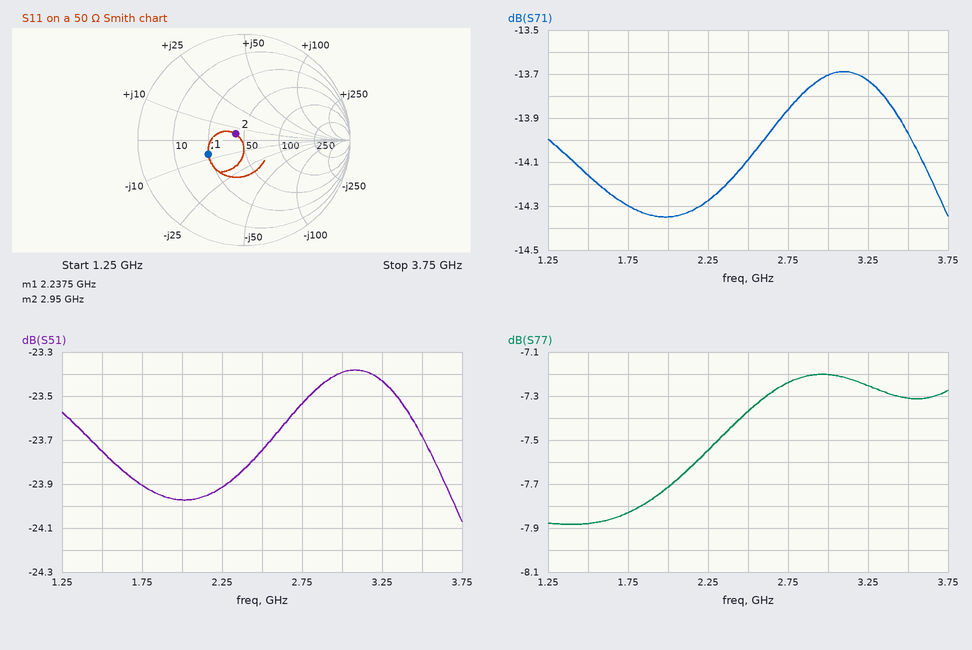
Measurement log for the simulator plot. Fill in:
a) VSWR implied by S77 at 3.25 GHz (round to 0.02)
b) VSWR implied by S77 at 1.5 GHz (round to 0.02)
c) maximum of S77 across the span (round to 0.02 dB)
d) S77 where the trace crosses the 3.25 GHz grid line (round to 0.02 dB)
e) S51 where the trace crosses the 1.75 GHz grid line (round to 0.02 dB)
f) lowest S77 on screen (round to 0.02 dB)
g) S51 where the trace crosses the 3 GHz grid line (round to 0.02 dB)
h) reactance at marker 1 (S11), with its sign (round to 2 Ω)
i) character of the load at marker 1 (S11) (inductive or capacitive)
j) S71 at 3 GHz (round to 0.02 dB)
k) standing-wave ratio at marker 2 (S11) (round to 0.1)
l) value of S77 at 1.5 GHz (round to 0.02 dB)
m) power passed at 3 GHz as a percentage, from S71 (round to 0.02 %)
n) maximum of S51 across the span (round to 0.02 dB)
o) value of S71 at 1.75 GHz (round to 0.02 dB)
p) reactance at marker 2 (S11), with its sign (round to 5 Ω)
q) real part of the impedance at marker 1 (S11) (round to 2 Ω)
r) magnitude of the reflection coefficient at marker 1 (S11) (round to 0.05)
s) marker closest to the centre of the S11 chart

2.54
2.36
-7.20 dB
-7.26 dB
-23.90 dB
-7.88 dB
-23.40 dB
-8 Ω
capacitive
-13.70 dB
1.2
-7.88 dB
4.26 %
-23.38 dB
-14.30 dB
+5 Ω
24 Ω
0.35
marker 2
